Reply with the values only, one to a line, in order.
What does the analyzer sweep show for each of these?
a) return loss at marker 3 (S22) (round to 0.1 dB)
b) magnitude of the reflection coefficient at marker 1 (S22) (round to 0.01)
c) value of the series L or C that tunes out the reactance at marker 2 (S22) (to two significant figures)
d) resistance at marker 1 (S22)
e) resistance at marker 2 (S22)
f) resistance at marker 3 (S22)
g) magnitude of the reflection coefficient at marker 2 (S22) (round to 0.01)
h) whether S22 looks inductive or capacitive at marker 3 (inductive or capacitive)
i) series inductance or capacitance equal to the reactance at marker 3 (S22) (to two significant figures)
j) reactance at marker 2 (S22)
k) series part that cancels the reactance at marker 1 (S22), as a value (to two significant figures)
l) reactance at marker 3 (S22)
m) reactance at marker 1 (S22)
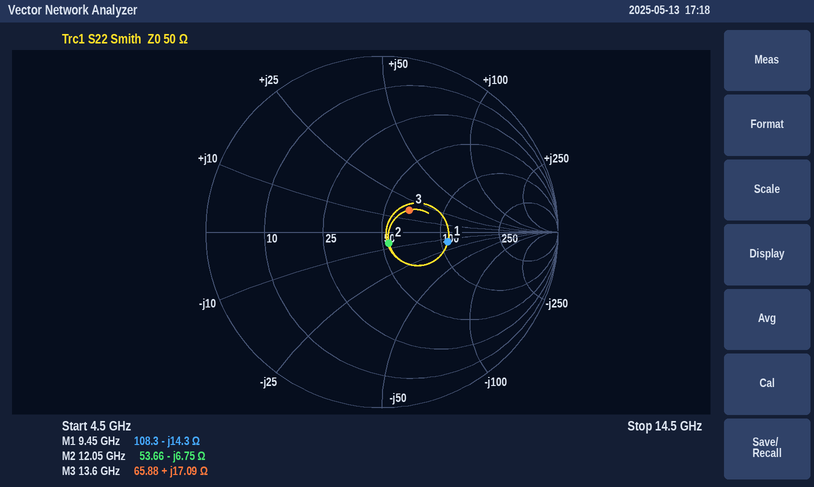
14.0 dB
0.38
89 pH
108.3 Ω
53.66 Ω
65.88 Ω
0.07
inductive
200 pH
-6.75 Ω
240 pH
+17.09 Ω
-14.3 Ω
